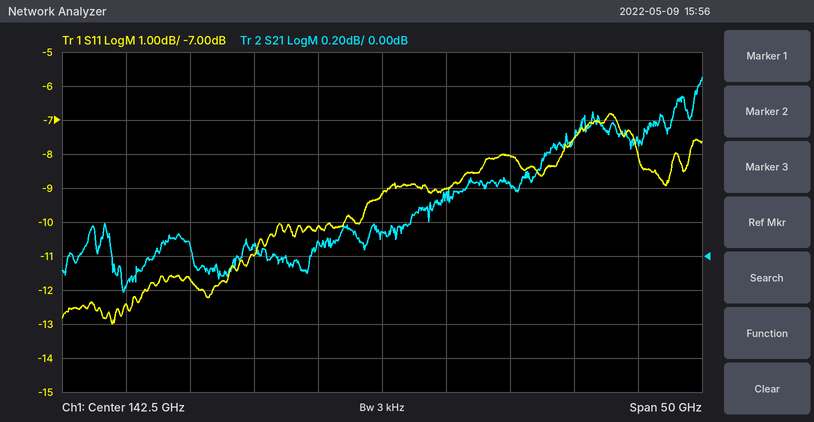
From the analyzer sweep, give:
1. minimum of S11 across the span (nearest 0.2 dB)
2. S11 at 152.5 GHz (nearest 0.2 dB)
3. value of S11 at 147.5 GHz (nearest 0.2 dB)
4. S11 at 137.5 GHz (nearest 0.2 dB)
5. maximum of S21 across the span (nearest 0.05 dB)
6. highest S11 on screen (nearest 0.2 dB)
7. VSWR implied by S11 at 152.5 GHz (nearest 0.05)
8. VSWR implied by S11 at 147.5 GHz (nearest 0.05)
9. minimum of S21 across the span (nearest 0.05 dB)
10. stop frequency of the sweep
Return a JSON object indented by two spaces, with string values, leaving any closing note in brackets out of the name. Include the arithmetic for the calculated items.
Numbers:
{
  "minimum of S11 across the span": "-13.0 dB",
  "S11 at 152.5 GHz": "-8.0 dB",
  "value of S11 at 147.5 GHz": "-9.0 dB",
  "S11 at 137.5 GHz": "-10.2 dB",
  "maximum of S21 across the span": "1.05 dB",
  "highest S11 on screen": "-6.8 dB",
  "VSWR implied by S11 at 152.5 GHz": "|Γ| = 10^(-8/20) = 0.3981; VSWR = (1 + 0.3981)/(1 − 0.3981) ≈ 2.32, so 2.30 to the nearest 0.05",
  "VSWR implied by S11 at 147.5 GHz": "|Γ| = 10^(-9/20) = 0.3548; VSWR = (1 + 0.3548)/(1 − 0.3548) ≈ 2.10",
  "minimum of S21 across the span": "-0.20 dB",
  "stop frequency of the sweep": "167.5 GHz"
}
